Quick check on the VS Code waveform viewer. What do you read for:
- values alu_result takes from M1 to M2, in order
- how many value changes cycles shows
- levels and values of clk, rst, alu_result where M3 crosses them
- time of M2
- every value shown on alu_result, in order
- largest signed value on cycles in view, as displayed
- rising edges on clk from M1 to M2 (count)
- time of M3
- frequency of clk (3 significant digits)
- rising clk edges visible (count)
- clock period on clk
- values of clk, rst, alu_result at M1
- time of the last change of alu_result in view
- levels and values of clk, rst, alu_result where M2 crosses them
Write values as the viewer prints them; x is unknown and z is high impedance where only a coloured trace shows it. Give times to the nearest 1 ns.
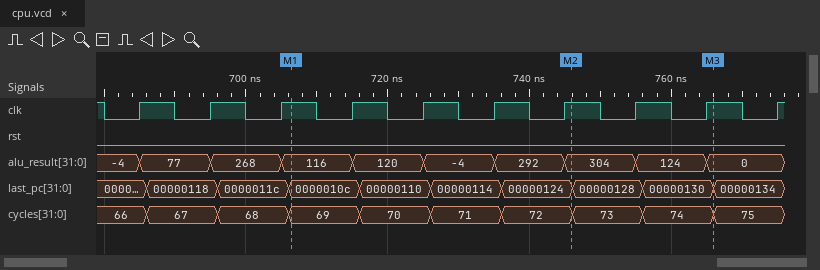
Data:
116, 120, -4, 292, 304
9
clk=1, rst=0, alu_result=0
746 ns
-4, 77, 268, 116, 120, -4, 292, 304, 124, 0
75
4
766 ns
100 MHz
10
10 ns
clk=1, rst=0, alu_result=116
765 ns
clk=1, rst=0, alu_result=304
